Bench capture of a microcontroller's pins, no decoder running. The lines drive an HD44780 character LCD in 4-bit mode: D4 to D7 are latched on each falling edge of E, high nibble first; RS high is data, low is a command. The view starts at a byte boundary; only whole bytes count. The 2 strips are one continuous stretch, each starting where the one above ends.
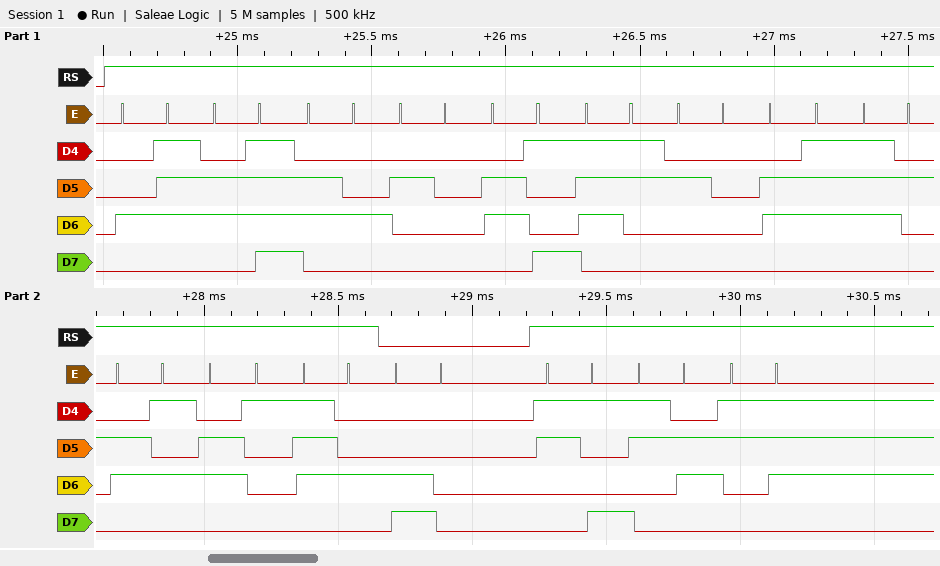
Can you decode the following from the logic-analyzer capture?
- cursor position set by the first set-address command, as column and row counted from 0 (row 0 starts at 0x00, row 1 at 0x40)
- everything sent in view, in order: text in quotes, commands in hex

column 0, row 1
"God is great" 0xC0 "967"
